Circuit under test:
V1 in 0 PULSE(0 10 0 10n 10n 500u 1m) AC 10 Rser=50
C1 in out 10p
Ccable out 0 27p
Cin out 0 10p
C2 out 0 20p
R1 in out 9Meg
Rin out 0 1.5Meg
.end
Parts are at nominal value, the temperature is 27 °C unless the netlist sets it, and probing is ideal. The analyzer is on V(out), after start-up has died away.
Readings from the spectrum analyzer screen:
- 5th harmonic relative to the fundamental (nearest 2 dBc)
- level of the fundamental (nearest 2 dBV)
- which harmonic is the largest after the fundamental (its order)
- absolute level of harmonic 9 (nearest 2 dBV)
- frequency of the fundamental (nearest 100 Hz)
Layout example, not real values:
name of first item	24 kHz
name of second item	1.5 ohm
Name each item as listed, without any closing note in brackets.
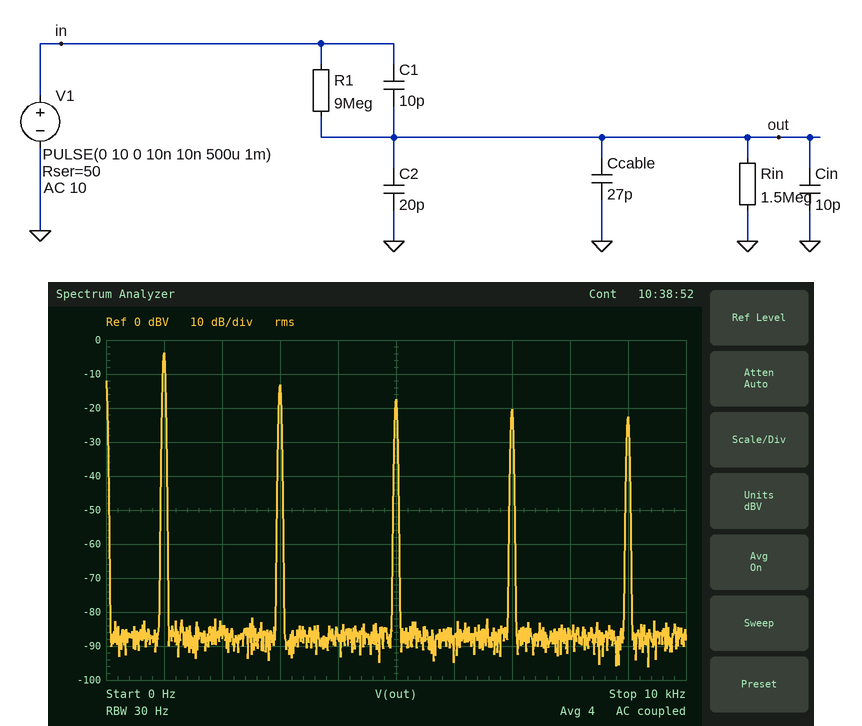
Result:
5th harmonic relative to the fundamental	-14 dBc
level of the fundamental	-4 dBV
which harmonic is the largest after the fundamental	3
absolute level of harmonic 9	-22 dBV
frequency of the fundamental	1.0 kHz
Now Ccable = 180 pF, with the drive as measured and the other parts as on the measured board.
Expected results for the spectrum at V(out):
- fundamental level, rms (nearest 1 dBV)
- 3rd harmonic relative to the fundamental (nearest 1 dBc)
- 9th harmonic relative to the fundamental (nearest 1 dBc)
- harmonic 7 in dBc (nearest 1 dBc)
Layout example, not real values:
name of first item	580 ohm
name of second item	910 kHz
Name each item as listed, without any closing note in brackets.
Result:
fundamental level, rms	-9 dBV
3rd harmonic relative to the fundamental	-13 dBc
9th harmonic relative to the fundamental	-24 dBc
harmonic 7 in dBc	-22 dBc
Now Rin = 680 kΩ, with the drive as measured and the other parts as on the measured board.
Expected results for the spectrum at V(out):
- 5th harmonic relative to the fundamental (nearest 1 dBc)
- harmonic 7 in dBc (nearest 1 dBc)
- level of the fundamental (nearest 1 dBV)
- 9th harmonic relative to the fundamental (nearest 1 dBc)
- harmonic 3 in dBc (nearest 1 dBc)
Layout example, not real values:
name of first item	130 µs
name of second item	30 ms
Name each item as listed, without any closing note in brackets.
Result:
5th harmonic relative to the fundamental	-10 dBc
harmonic 7 in dBc	-12 dBc
level of the fundamental	-9 dBV
9th harmonic relative to the fundamental	-14 dBc
harmonic 3 in dBc	-7 dBc
